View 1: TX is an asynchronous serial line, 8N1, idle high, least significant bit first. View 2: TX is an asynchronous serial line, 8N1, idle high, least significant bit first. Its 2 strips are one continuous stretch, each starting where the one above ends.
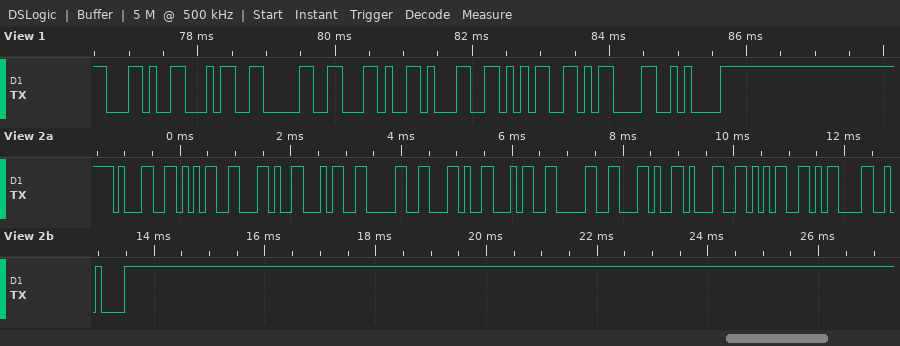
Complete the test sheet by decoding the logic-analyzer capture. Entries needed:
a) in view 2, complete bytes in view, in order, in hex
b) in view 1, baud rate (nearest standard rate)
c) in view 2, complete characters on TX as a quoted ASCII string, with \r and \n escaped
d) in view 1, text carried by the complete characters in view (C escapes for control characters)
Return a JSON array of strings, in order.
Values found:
["31 35 2C 34 30 2C 34 30 2C 31 35 0D 0A", "9600 baud", "\"15,40,40,15\\r\\n\"", "\",40,15\\r\\n\""]
